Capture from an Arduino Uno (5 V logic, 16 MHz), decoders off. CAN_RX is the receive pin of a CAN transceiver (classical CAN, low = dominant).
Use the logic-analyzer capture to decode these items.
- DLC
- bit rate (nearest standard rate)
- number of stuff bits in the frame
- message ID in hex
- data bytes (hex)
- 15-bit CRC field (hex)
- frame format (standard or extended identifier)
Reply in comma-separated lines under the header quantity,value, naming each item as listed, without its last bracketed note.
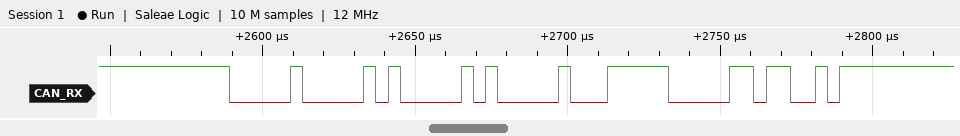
quantity,value
DLC,1
bit rate,250 kbit/s
number of stuff bits in the frame,6
message ID in hex,0x001
data bytes,00
15-bit CRC field,0x7C2C
frame format,standard
